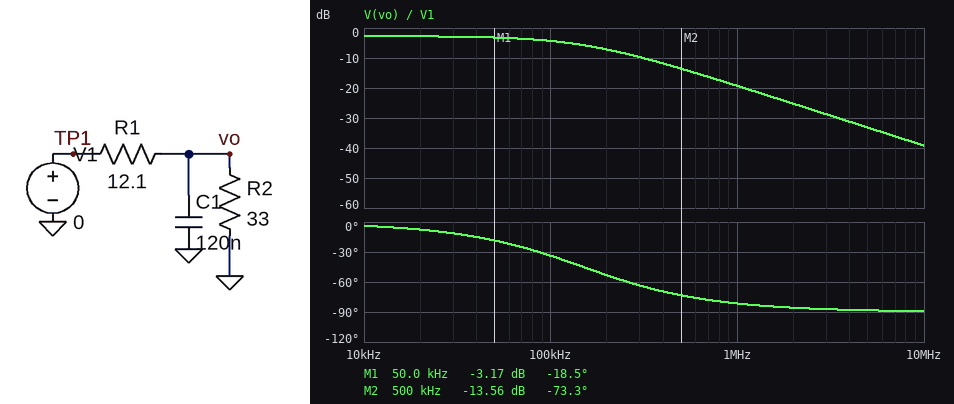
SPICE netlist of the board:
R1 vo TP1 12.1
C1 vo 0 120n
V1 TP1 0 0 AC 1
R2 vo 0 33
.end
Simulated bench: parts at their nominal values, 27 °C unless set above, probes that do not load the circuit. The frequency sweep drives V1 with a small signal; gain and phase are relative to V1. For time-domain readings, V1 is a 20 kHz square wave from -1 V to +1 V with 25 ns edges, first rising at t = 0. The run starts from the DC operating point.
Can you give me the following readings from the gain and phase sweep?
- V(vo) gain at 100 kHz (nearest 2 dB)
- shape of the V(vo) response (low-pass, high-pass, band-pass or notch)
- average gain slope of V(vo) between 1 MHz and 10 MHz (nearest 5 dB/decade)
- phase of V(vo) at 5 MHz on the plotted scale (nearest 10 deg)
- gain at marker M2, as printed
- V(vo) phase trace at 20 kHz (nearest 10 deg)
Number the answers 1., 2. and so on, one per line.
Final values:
1. -4 dB
2. low-pass
3. -20 dB/decade
4. -90 deg
5. -13.56 dB
6. -10 deg
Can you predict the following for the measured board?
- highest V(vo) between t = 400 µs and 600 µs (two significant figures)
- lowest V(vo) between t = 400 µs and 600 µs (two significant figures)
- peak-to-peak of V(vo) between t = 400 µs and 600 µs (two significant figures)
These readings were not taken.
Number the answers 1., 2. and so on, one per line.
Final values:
1. 730 mV
2. -730 mV
3. 1.5 V
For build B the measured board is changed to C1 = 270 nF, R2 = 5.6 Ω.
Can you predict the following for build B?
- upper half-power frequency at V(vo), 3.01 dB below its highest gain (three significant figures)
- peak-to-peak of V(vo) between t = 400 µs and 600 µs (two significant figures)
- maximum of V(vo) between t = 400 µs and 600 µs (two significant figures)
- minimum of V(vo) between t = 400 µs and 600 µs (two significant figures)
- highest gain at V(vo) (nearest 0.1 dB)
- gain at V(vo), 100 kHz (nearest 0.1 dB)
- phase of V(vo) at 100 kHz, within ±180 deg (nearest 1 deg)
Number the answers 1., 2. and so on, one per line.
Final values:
1. 154 kHz
2. 630 mV
3. 320 mV
4. -320 mV
5. -10.0 dB
6. -11.5 dB
7. -33 deg
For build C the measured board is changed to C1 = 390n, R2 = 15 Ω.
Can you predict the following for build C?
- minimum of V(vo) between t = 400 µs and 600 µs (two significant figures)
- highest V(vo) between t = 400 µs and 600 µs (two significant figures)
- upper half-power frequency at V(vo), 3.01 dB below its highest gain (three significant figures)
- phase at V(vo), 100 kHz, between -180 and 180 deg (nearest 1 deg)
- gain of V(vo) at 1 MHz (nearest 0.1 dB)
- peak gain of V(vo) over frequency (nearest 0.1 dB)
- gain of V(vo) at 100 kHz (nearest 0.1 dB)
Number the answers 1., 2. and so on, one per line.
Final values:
1. -550 mV
2. 550 mV
3. 60.9 kHz
4. -59 deg
5. -29.5 dB
6. -5.1 dB
7. -10.8 dB
